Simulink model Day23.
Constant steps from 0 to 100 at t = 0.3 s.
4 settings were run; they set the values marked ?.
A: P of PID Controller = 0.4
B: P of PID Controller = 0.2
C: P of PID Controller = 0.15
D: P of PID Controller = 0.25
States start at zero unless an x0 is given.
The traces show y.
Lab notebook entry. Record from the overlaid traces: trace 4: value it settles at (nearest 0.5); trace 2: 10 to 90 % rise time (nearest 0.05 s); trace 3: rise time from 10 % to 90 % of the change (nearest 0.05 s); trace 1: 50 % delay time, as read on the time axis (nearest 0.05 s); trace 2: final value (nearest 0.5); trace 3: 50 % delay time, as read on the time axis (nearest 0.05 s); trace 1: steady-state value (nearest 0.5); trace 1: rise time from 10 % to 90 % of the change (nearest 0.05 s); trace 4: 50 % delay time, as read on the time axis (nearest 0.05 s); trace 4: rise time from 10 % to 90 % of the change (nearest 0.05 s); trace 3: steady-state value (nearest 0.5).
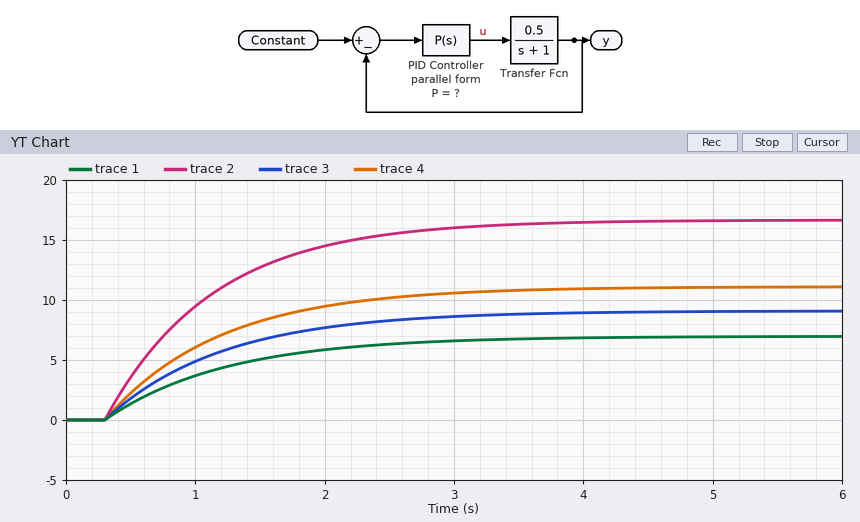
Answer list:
11.0
1.85 s
2.00 s
0.95 s
16.5
0.95 s
7.0
2.05 s
0.90 s
1.95 s
9.0
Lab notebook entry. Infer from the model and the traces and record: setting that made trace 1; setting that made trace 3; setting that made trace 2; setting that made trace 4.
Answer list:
C
B
A
D
